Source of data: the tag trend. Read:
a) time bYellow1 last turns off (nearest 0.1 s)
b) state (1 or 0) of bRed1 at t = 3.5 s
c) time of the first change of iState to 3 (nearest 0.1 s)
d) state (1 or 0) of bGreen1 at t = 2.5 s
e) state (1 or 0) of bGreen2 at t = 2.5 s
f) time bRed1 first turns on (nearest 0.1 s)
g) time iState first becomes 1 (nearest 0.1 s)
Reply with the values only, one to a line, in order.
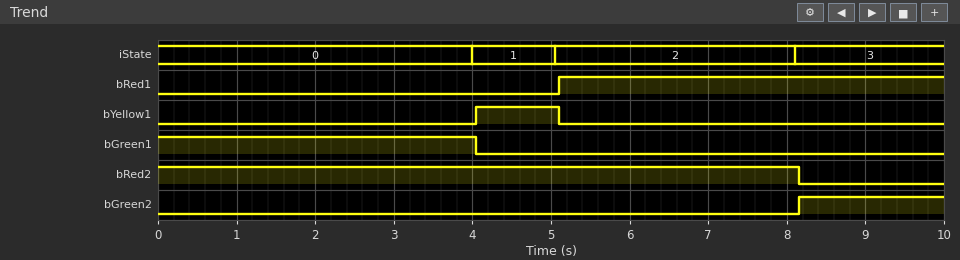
5.1 s
0
8.1 s
1
0
5.1 s
4.0 s
